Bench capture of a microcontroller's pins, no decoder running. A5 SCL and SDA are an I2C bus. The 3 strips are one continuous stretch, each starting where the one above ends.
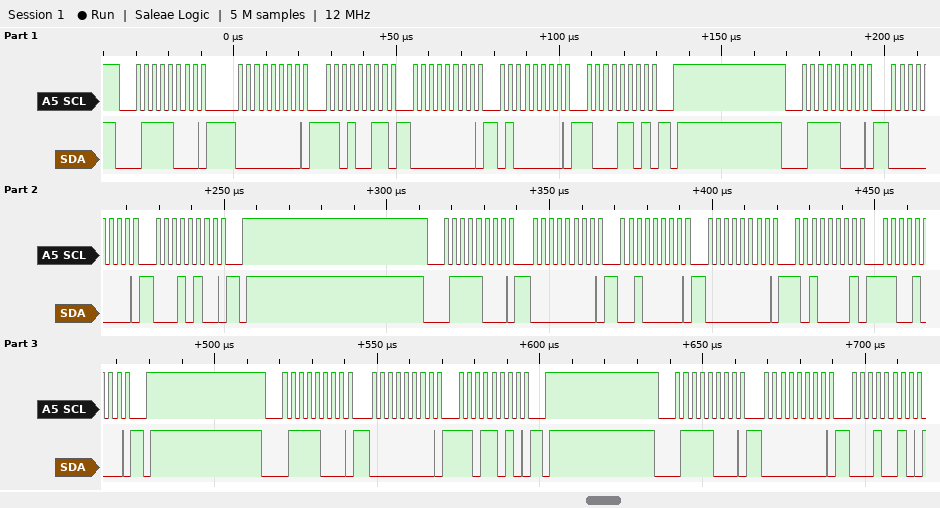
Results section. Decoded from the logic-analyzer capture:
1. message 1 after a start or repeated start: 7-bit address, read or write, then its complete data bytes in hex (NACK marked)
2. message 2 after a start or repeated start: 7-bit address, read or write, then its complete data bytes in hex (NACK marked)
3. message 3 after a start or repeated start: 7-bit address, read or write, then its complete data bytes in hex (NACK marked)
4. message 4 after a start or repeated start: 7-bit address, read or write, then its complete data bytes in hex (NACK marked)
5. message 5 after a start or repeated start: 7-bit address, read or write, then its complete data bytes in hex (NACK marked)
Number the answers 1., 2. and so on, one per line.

1. 0x3C write: 00 D3 00 40 8D
2. 0x3C write: 00 14
3. 0x3C write: 00 20 00 A1 C8
4. 0x3C write: 00 DA
5. 0x3C write: 00 12
